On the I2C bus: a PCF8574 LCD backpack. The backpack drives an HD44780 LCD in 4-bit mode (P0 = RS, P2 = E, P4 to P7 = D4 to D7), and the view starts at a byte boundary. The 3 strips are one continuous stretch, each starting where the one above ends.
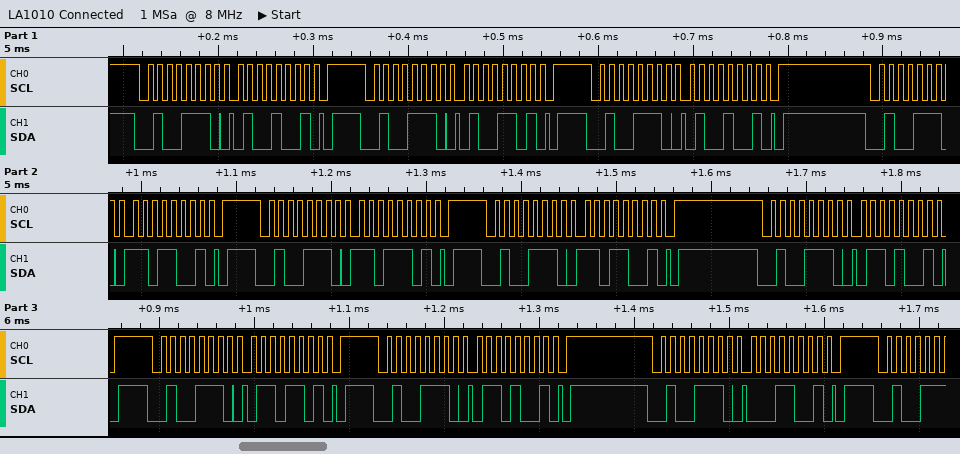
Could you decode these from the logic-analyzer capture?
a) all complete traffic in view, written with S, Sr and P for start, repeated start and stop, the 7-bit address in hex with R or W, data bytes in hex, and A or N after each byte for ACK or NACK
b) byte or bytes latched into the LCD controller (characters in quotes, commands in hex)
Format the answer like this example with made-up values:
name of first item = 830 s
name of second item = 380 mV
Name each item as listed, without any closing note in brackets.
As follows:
all complete traffic in view, written with S, Sr and P for start, repeated start and stop, the 7-bit address in hex with R or W, data bytes in hex, and A or N after each byte for ACK or NACK = S 27W A 49 A P S 27W A 4D A P S 27W A 49 A P S 27W A D9 A P S 27W A DD A P S 27W A D9 A P S 27W A 69 A P S 27W A 6D A P S 27W A 69 A P S 27W A 19 A P
byte or bytes latched into the LCD controller = 'M'
